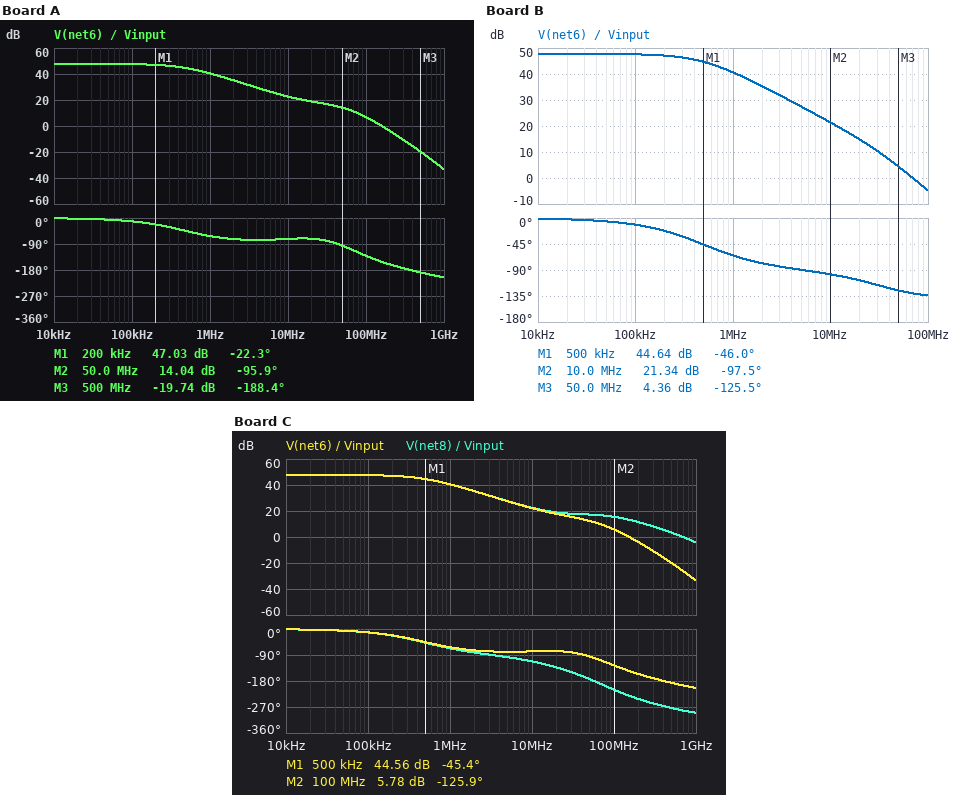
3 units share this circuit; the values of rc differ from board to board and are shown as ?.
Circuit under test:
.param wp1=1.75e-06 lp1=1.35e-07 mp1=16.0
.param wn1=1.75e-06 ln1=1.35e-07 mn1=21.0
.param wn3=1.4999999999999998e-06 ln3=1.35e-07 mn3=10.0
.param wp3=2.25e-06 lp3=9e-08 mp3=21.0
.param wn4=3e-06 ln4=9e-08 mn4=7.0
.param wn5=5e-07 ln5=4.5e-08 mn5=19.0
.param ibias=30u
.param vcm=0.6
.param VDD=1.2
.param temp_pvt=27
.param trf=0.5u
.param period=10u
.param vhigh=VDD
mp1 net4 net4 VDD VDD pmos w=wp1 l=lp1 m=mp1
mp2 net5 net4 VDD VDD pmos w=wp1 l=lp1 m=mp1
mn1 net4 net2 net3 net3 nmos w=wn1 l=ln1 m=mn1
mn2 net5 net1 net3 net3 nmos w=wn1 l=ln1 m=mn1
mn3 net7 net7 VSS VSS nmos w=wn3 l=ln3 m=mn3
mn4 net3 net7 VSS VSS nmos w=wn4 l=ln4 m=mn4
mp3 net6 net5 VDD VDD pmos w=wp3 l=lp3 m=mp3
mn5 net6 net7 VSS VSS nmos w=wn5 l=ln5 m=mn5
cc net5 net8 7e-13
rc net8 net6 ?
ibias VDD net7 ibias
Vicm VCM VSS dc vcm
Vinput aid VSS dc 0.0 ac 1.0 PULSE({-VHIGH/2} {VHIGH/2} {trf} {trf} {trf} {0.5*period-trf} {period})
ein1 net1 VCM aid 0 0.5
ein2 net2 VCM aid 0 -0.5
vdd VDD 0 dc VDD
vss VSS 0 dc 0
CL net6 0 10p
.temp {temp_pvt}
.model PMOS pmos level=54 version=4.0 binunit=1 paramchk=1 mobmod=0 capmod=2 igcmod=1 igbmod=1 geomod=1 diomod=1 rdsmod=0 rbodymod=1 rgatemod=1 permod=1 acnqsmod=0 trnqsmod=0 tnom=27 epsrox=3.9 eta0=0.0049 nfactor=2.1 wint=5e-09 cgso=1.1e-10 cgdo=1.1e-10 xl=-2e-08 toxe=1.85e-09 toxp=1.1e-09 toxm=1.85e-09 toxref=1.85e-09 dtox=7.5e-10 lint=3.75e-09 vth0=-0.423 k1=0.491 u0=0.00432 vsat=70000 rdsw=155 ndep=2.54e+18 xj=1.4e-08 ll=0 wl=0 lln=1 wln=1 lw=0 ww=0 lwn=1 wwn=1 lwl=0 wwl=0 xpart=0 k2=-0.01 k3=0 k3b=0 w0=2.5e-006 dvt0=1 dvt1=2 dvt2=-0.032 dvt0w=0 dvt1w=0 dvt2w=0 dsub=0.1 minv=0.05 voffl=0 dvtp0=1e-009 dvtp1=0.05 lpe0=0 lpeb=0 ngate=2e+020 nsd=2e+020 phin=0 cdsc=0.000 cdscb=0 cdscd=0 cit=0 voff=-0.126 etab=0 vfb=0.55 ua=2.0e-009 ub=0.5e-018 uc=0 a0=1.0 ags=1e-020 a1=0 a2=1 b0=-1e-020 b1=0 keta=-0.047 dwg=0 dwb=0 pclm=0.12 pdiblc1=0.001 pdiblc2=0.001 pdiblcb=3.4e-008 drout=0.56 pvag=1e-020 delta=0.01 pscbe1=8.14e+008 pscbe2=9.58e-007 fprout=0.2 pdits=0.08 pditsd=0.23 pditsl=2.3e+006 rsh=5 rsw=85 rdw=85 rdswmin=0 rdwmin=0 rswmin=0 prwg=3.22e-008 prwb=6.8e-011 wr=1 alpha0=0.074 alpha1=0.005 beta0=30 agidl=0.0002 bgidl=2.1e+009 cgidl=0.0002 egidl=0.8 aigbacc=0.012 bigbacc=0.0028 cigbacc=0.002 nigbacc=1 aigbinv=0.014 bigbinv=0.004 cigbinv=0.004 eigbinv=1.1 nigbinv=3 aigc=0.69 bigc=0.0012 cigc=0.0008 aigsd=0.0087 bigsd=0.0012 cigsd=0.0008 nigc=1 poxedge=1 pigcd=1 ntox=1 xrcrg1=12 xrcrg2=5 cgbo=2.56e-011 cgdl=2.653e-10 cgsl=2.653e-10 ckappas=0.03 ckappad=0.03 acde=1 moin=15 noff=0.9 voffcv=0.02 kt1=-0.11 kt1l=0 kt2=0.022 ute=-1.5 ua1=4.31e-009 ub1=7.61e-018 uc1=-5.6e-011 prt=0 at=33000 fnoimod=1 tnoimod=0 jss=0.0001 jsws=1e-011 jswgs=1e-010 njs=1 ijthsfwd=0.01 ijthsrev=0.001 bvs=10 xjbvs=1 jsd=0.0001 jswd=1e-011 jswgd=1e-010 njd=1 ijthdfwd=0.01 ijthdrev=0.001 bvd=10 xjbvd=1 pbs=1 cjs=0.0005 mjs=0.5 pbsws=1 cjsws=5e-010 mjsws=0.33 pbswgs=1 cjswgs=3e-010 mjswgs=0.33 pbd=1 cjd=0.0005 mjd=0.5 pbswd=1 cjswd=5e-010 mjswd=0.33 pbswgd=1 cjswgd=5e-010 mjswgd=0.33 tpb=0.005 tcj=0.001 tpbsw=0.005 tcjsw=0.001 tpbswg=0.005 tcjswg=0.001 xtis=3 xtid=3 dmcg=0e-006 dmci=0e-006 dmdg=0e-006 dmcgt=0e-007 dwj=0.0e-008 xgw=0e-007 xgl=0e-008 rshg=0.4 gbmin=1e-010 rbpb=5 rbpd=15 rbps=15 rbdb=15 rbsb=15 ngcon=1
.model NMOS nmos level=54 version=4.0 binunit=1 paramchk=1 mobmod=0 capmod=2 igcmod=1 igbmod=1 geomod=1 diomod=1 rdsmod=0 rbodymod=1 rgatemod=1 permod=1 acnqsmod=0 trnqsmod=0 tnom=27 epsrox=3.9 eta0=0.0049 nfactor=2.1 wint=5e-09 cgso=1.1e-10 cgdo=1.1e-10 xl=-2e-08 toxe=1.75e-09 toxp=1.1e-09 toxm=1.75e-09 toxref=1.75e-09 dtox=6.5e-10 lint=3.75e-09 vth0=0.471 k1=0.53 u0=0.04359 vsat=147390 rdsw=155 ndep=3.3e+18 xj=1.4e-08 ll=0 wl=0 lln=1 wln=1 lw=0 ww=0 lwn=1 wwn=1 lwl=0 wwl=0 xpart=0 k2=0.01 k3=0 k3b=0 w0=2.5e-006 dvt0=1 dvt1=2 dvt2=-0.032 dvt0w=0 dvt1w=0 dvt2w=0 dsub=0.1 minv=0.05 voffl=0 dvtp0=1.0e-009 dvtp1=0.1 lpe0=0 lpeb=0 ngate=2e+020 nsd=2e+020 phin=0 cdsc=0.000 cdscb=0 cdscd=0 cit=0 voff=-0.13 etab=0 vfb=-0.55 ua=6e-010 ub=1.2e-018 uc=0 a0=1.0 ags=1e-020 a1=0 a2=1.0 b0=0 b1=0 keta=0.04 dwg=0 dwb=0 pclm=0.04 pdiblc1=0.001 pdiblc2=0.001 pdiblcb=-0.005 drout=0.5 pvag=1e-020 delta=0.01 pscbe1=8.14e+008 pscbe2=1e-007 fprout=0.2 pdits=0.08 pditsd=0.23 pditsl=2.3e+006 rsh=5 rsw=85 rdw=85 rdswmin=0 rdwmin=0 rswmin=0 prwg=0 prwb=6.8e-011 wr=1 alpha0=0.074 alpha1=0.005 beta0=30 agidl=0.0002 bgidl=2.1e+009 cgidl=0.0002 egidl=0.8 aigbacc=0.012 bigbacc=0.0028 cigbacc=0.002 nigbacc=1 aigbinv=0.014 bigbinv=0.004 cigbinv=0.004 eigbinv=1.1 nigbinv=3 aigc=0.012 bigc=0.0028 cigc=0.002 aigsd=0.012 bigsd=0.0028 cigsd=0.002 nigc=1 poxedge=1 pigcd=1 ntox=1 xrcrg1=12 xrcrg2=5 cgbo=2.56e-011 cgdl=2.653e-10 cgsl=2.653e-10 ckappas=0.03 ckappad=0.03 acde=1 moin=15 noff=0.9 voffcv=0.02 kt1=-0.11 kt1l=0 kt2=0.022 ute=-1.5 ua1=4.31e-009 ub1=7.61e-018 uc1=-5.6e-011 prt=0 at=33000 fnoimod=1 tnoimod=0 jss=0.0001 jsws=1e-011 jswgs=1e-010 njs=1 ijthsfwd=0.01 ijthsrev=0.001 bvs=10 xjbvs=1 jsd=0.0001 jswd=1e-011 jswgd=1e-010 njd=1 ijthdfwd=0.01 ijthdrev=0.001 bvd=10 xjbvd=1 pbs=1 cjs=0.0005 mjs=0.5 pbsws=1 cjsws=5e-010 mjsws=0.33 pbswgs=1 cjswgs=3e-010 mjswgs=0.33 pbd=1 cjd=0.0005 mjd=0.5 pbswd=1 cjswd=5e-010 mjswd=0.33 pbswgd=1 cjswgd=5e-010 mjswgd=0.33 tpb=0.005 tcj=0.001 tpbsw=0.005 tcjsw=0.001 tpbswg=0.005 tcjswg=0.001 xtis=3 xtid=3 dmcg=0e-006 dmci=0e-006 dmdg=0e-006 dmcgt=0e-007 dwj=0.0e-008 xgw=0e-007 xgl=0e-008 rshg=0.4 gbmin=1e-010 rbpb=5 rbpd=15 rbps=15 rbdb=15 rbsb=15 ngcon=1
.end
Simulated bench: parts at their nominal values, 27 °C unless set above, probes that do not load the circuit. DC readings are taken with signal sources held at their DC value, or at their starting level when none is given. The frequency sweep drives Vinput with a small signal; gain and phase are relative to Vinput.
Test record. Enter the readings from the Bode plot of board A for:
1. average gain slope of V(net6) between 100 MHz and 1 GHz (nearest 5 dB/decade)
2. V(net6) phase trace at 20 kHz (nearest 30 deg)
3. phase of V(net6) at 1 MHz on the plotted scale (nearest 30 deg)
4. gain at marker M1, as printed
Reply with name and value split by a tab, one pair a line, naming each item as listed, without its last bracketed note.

average gain slope of V(net6) between 100 MHz and 1 GHz	-40 dB/decade
V(net6) phase trace at 20 kHz	0 deg
phase of V(net6) at 1 MHz on the plotted scale	-60 deg
gain at marker M1, as printed	47.03 dB
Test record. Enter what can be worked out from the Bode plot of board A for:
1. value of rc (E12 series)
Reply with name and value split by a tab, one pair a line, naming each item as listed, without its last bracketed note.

value of rc	15 kΩ
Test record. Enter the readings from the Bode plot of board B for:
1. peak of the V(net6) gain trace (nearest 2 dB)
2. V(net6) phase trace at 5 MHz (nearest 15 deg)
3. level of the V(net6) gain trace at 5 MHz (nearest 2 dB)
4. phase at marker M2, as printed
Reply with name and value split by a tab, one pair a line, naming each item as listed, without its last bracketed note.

peak of the V(net6) gain trace	48 dB
V(net6) phase trace at 5 MHz	-90 deg
level of the V(net6) gain trace at 5 MHz	28 dB
phase at marker M2, as printed	-97.5 deg
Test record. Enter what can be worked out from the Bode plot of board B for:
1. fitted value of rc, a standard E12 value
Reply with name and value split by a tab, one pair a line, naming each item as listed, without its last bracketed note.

fitted value of rc, a standard E12 value	2.2 kΩ
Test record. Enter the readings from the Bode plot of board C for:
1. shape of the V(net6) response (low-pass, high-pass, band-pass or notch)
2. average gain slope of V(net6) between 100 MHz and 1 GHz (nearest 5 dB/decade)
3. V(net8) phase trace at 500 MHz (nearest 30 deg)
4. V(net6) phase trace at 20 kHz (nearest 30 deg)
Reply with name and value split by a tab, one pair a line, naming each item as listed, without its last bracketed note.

shape of the V(net6) response	low-pass
average gain slope of V(net6) between 100 MHz and 1 GHz	-40 dB/decade
V(net8) phase trace at 500 MHz	-270 deg
V(net6) phase trace at 20 kHz	0 deg
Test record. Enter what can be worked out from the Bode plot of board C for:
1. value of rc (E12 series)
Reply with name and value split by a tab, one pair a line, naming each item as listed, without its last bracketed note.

value of rc	12 kΩ
